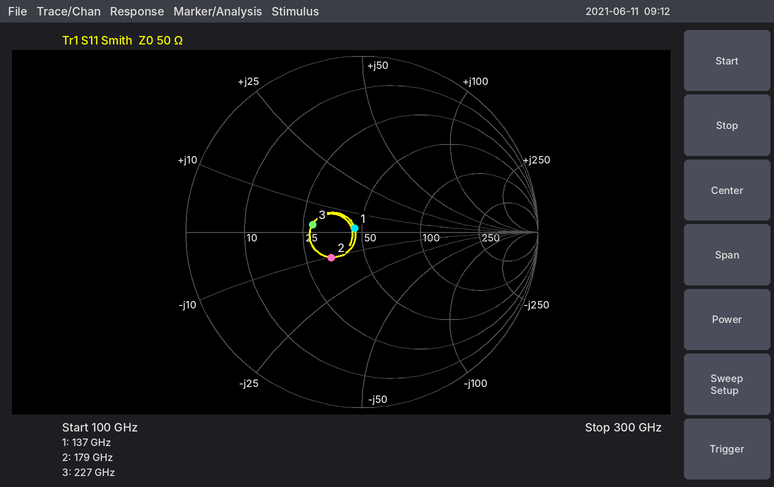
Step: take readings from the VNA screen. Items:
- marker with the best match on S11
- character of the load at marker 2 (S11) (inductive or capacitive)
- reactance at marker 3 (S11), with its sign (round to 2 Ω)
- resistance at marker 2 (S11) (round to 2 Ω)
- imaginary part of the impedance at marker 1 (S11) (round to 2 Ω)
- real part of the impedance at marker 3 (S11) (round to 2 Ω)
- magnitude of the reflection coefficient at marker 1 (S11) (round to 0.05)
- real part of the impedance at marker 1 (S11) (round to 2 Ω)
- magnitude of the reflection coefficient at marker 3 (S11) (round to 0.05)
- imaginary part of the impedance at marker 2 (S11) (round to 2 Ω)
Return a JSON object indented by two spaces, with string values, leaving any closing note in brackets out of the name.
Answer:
{
  "marker with the best match on S11": "marker 1",
  "character of the load at marker 2 (S11)": "capacitive",
  "reactance at marker 3 (S11), with its sign": "+2 Ω",
  "resistance at marker 2 (S11)": "34 Ω",
  "imaginary part of the impedance at marker 1 (S11)": "+2 Ω",
  "real part of the impedance at marker 3 (S11)": "28 Ω",
  "magnitude of the reflection coefficient at marker 1 (S11)": "0.05",
  "real part of the impedance at marker 1 (S11)": "46 Ω",
  "magnitude of the reflection coefficient at marker 3 (S11)": "0.30",
  "imaginary part of the impedance at marker 2 (S11)": "-10 Ω"
}
